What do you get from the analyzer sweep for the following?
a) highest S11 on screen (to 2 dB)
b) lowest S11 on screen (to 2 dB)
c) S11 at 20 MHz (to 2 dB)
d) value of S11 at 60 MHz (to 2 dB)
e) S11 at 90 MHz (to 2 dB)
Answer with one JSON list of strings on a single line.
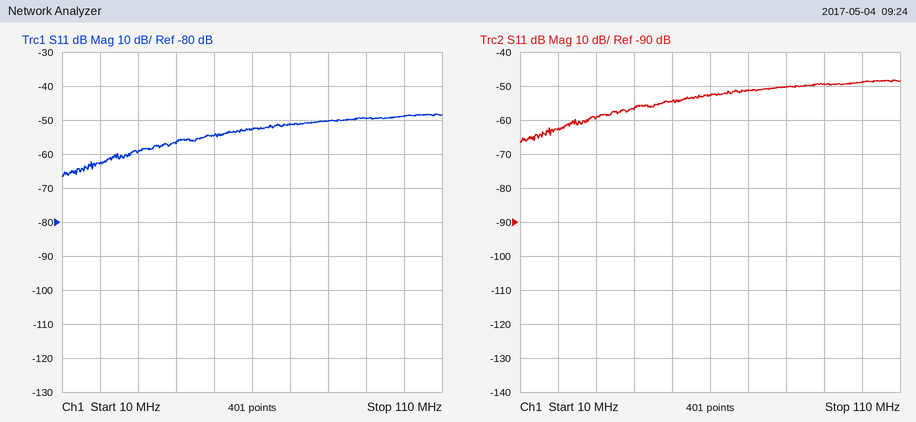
["-48 dB", "-66 dB", "-62 dB", "-52 dB", "-50 dB"]
